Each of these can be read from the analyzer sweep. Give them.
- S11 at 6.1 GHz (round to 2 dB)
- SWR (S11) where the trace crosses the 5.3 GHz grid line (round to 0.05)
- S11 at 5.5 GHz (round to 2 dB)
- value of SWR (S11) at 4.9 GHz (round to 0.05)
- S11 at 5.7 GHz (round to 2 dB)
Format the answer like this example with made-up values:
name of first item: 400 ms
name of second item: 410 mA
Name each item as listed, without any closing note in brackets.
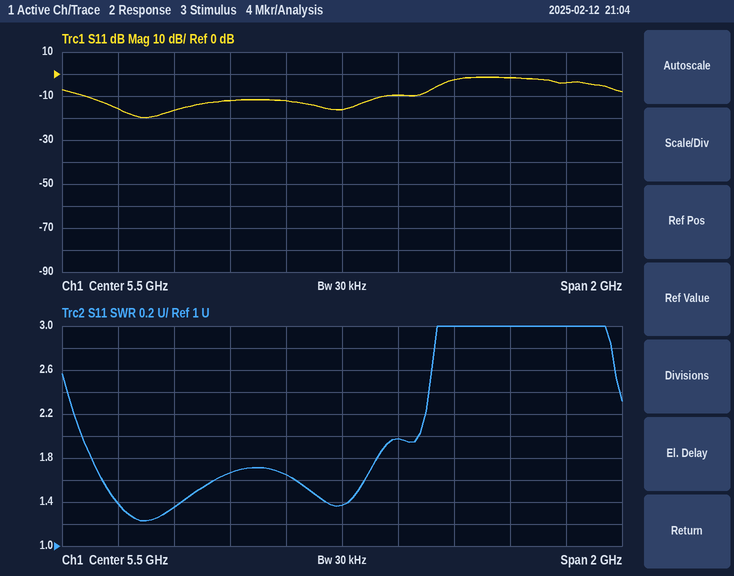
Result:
S11 at 6.1 GHz: -2 dB
SWR (S11) where the trace crosses the 5.3 GHz grid line: 1.65
S11 at 5.5 GHz: -16 dB
value of SWR (S11) at 4.9 GHz: 1.35
S11 at 5.7 GHz: -10 dB
